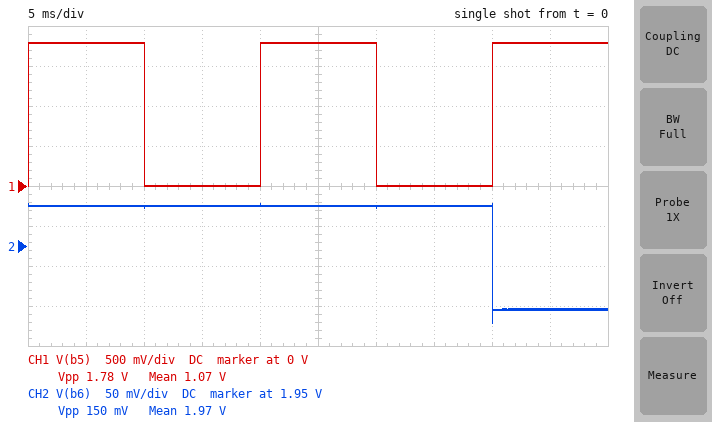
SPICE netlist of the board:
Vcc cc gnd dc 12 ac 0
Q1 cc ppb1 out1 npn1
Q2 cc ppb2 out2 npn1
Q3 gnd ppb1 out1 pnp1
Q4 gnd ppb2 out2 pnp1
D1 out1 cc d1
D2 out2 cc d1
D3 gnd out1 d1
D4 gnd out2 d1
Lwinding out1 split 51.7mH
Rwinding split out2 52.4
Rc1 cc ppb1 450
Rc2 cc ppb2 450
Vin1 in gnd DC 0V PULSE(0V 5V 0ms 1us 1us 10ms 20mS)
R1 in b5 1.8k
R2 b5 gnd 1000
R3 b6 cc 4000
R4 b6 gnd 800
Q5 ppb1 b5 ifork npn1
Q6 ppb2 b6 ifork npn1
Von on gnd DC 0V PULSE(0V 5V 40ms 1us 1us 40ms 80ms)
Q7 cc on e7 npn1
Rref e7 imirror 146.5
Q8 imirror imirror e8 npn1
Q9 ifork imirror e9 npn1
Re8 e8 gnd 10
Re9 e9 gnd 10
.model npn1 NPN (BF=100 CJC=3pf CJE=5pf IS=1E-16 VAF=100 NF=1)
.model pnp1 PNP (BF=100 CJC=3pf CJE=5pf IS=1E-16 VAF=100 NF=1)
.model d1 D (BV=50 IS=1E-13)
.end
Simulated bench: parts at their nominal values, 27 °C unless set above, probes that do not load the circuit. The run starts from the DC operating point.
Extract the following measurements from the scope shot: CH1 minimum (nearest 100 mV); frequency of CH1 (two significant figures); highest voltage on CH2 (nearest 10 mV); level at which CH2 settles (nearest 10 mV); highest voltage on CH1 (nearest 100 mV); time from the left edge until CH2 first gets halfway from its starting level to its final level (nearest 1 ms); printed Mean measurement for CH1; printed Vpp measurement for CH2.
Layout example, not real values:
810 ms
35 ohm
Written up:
0 V
50 Hz
2.00 V
1.87 V
1.8 V
40 ms
1.07 V
150 mV
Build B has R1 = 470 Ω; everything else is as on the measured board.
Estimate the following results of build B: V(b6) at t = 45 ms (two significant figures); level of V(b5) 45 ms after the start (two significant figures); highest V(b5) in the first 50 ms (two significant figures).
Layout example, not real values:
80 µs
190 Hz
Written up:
2.0 V
3.3 V
3.4 V
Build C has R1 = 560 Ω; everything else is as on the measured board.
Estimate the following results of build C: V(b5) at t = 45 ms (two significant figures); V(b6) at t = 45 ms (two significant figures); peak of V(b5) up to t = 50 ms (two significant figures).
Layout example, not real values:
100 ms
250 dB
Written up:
3.1 V
2.0 V
3.2 V
